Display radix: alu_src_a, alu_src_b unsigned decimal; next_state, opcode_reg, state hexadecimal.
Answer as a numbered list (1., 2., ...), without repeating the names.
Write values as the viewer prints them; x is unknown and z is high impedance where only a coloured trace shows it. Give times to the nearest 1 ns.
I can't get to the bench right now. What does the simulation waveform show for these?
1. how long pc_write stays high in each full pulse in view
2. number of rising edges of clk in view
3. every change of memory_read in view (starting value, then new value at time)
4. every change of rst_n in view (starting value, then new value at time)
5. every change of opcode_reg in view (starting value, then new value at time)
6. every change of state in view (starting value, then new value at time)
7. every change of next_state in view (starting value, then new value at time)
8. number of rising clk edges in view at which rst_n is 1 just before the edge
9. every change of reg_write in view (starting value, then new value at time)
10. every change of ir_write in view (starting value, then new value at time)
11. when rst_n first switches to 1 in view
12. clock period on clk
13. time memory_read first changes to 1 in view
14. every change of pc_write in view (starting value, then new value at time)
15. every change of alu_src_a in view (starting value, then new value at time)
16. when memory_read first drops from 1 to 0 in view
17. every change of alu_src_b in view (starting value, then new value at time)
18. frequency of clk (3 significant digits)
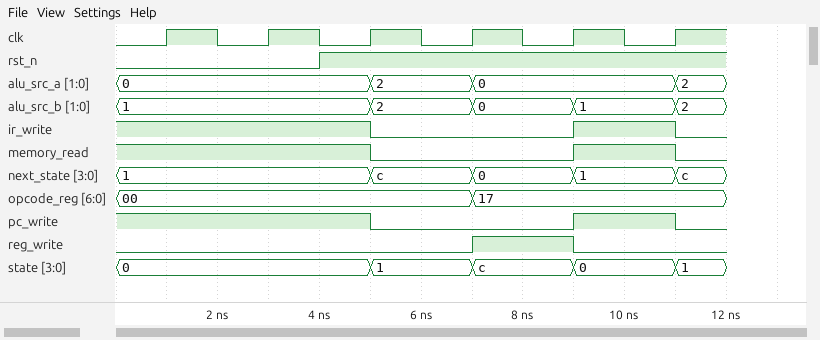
1. 2 ns
2. 6
3. 1, 0 at 5 ns, 1 at 9 ns, 0 at 11 ns
4. 0, 1 at 4 ns
5. 00, 17 at 7 ns
6. 0, 1 at 5 ns, c at 7 ns, 0 at 9 ns, 1 at 11 ns
7. 1, c at 5 ns, 0 at 7 ns, 1 at 9 ns, c at 11 ns
8. 4
9. 0, 1 at 7 ns, 0 at 9 ns
10. 1, 0 at 5 ns, 1 at 9 ns, 0 at 11 ns
11. 4 ns
12. 2 ns
13. 9 ns
14. 1, 0 at 5 ns, 1 at 9 ns, 0 at 11 ns
15. 0, 2 at 5 ns, 0 at 7 ns, 2 at 11 ns
16. 5 ns
17. 1, 2 at 5 ns, 0 at 7 ns, 1 at 9 ns, 2 at 11 ns
18. 500 MHz
